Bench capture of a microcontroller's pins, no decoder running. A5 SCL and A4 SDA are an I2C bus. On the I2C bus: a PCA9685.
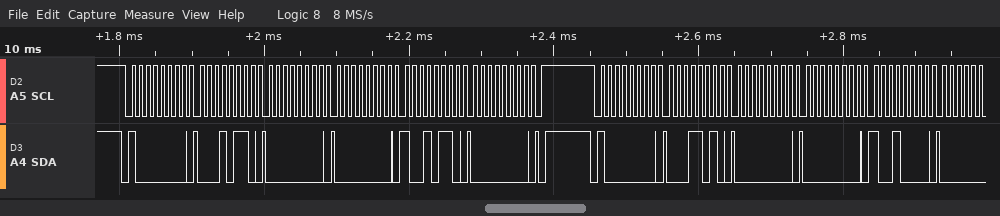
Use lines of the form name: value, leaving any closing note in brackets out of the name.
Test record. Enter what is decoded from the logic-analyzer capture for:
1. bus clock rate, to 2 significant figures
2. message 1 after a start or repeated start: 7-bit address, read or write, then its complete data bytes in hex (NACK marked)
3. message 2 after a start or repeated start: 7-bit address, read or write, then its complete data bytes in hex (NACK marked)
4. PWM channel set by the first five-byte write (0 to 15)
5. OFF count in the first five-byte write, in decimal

bus clock rate, to 2 significant figures: 100 kHz
message 1 after a start or repeated start: 7-bit address, read or write, then its complete data bytes in hex: 0x40 write: 16 00 00 96 00
message 2 after a start or repeated start: 7-bit address, read or write, then its complete data bytes in hex: 0x40 write: 1A 00 00 90
PWM channel set by the first five-byte write: 4
OFF count in the first five-byte write, in decimal: 150
